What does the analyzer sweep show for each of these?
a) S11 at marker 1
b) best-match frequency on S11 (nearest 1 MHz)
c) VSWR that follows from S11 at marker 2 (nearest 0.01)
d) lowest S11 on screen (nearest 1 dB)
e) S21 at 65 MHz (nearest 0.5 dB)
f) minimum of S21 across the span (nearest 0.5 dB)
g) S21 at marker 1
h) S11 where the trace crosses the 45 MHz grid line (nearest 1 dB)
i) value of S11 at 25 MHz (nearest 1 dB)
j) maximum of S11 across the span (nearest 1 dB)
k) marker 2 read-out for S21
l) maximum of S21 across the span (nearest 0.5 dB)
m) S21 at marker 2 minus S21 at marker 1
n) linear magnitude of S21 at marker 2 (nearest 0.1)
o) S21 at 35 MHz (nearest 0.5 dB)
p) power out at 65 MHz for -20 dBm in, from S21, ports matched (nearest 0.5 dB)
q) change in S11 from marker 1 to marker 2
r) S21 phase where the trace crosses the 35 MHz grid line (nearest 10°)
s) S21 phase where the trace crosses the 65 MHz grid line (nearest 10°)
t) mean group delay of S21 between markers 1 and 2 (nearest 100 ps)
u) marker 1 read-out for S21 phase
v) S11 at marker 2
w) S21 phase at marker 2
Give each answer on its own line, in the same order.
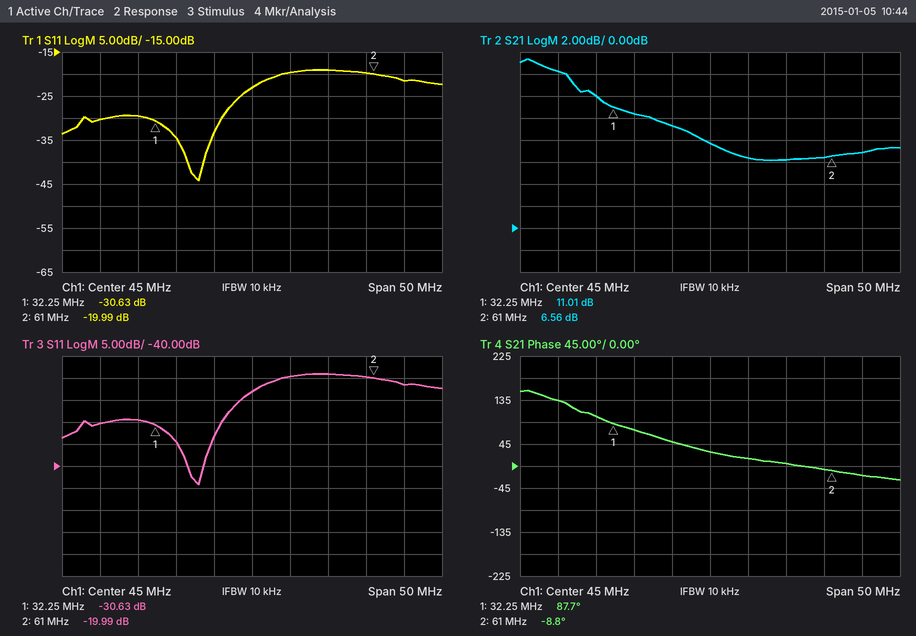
-30.63 dB
38 MHz
1.22
-44 dB
7.0 dB
6.0 dB
11.01 dB
-23 dB
-30 dB
-19 dB
6.56 dB
15.5 dB
-4.45 dB
2.1
10.5 dB
-13.0 dBm
10.64 dB
70°
-20°
9.3 ns
87.7°
-19.99 dB
-8.8°
